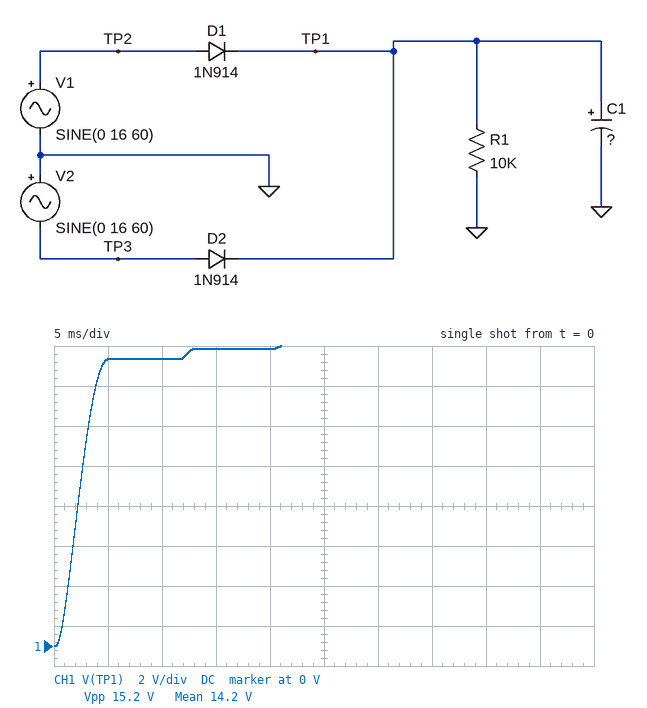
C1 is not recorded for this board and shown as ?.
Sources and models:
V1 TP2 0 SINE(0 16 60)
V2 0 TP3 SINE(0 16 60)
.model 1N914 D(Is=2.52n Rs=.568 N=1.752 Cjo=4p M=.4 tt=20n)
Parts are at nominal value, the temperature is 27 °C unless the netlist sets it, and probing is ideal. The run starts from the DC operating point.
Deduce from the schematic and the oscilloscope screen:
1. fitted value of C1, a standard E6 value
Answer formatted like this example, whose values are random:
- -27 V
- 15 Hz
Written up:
- 1.5 mF
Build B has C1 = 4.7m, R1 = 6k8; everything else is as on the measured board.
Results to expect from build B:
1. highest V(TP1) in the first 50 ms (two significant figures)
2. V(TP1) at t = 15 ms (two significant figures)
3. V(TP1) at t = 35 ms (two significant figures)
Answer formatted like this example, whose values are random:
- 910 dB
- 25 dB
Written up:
- 15 V
- 13 V
- 14 V
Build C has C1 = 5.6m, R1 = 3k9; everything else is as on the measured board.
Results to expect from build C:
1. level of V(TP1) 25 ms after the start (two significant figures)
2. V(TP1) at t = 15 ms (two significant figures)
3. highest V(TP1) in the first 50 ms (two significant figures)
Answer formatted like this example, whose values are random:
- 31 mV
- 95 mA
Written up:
- 14 V
- 13 V
- 15 V
